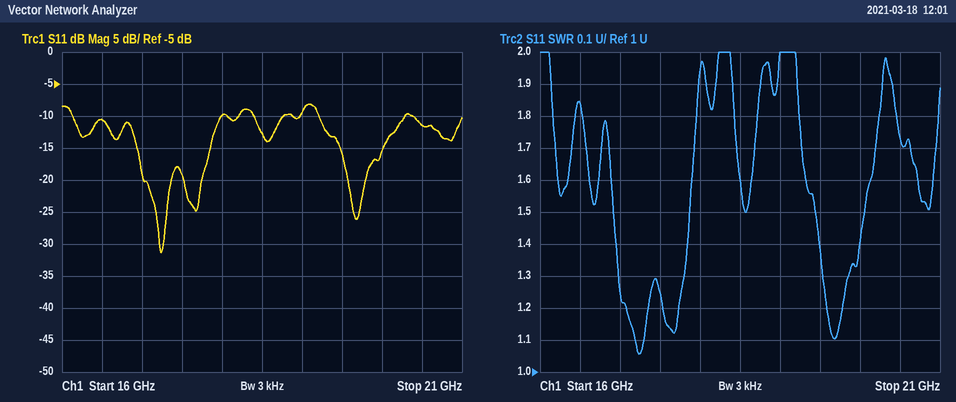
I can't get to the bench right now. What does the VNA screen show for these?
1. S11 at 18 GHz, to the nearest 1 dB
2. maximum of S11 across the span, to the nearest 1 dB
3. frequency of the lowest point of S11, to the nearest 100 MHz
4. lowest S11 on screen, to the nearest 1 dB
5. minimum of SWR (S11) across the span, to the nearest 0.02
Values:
-10 dB
-8 dB
17.2 GHz
-31 dB
1.06
